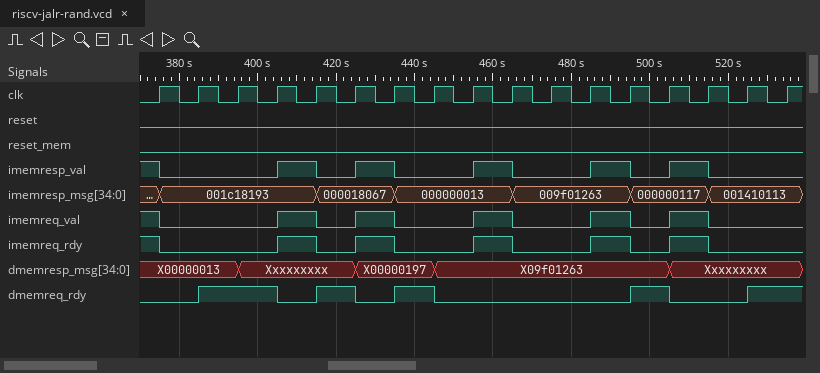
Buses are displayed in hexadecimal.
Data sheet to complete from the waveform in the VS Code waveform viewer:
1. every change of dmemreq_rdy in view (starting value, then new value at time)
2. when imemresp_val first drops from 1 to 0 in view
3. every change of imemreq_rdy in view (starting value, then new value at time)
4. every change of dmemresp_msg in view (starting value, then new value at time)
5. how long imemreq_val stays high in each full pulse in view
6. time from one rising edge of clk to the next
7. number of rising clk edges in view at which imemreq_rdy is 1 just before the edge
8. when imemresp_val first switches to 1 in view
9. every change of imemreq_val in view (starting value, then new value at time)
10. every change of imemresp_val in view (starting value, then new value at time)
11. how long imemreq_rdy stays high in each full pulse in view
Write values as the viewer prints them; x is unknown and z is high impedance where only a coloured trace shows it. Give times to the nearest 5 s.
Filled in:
0, 1 at 385 s, 0 at 405 s, 1 at 415 s, 0 at 425 s, 1 at 435 s, 0 at 445 s, 1 at 495 s, 0 at 505 s, 1 at 525 s
375 s
1, 0 at 375 s, 1 at 405 s, 0 at 415 s, 1 at 425 s, 0 at 435 s, 1 at 455 s, 0 at 465 s, 1 at 485 s, 0 at 495 s, 1 at 505 s, 0 at 515 s
X00000013, Xxxxxxxxx at 395 s, X00000197 at 425 s, X09f01263 at 445 s, Xxxxxxxxx at 505 s
10 s, 10 s, 10 s, 10 s, 10 s
10 s
6
405 s
1, 0 at 375 s, 1 at 405 s, 0 at 415 s, 1 at 425 s, 0 at 435 s, 1 at 455 s, 0 at 465 s, 1 at 485 s, 0 at 495 s, 1 at 505 s, 0 at 515 s
1, 0 at 375 s, 1 at 405 s, 0 at 415 s, 1 at 425 s, 0 at 435 s, 1 at 455 s, 0 at 465 s, 1 at 485 s, 0 at 495 s, 1 at 505 s, 0 at 515 s
10 s, 10 s, 10 s, 10 s, 10 s
